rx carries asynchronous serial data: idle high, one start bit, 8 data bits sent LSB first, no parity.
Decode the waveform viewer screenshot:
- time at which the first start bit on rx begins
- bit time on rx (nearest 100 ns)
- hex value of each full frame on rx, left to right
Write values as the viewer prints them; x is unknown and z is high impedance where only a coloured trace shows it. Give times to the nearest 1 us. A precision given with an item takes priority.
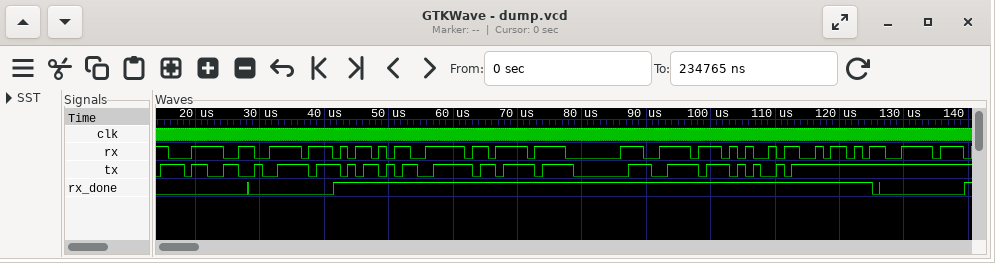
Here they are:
16 us
1200 ns
3C, DE, AD, BE, EF, C0, DE, A5, 5A, DE
